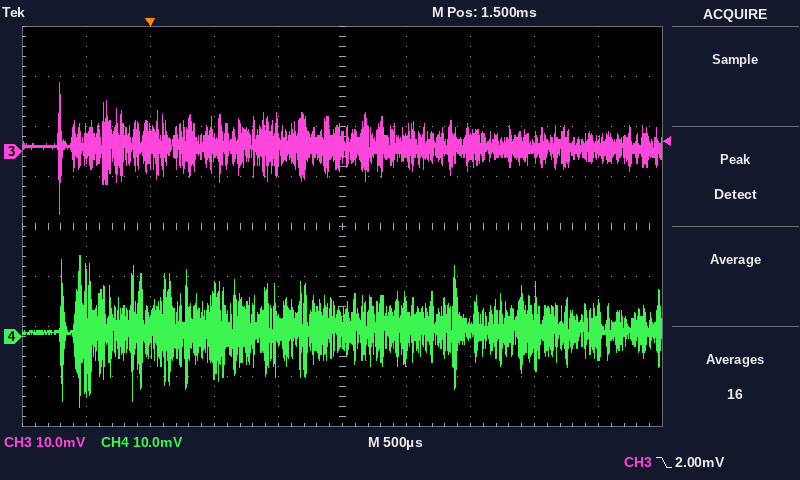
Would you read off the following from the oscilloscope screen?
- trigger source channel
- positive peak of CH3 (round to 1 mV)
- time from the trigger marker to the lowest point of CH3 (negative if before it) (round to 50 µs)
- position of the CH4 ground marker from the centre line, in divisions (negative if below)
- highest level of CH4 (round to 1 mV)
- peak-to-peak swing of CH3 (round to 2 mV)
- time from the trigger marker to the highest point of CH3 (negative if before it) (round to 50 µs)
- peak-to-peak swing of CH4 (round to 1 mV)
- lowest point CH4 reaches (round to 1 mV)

CH3
14 mV
-700 µs
-2.2 div
16 mV
26 mV
-700 µs
30 mV
-14 mV
